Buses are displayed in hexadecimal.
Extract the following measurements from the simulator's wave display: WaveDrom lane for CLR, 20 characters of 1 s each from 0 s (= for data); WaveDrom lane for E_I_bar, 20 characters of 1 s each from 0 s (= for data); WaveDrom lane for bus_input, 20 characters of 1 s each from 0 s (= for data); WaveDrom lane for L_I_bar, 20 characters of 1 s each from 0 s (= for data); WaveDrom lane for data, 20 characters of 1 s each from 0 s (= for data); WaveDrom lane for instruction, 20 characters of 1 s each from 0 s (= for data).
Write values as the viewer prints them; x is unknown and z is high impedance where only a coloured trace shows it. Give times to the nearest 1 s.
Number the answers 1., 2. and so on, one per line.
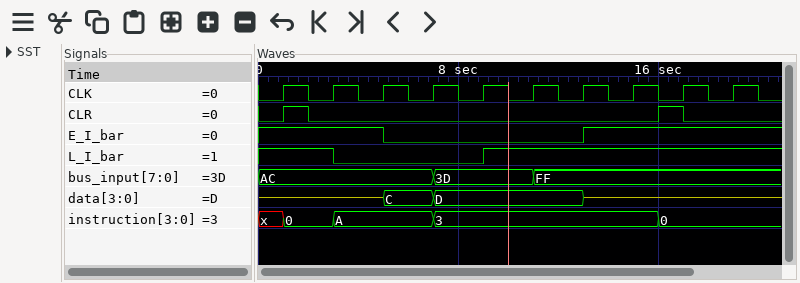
1. {name: 'CLR', wave: '010.............10..'}
2. {name: 'E_I_bar', wave: '1....0.......1......'}
3. {name: 'bus_input', wave: '=......=...=........', data: 'AC 3D FF'}
4. {name: 'L_I_bar', wave: '1..0.....1..........'}
5. {name: 'data', wave: 'z....=.=.....z......', data: 'C D'}
6. {name: 'instruction', wave: 'x=.=...=........=...', data: '0 A 3 0'}
